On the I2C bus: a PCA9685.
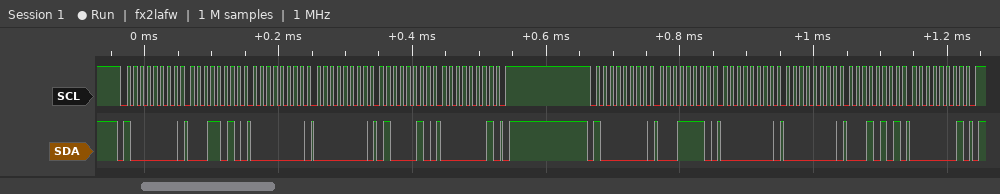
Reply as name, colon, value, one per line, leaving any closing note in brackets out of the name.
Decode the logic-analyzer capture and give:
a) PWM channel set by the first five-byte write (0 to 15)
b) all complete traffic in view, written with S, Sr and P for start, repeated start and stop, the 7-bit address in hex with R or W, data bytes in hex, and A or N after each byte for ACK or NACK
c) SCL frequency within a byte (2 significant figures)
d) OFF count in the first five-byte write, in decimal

PWM channel set by the first five-byte write: 5
all complete traffic in view, written with S, Sr and P for start, repeated start and stop, the 7-bit address in hex with R or W, data bytes in hex, and A or N after each byte for ACK or NACK: S 40W A 1A A 00 A 00 A 42 A 01 A P S 40W A 1E A 00 A 00 A 15 A 01 A P
SCL frequency within a byte: 100 kHz
OFF count in the first five-byte write, in decimal: 322
